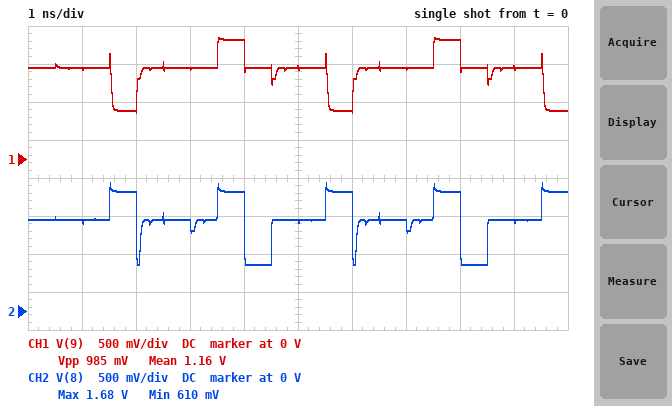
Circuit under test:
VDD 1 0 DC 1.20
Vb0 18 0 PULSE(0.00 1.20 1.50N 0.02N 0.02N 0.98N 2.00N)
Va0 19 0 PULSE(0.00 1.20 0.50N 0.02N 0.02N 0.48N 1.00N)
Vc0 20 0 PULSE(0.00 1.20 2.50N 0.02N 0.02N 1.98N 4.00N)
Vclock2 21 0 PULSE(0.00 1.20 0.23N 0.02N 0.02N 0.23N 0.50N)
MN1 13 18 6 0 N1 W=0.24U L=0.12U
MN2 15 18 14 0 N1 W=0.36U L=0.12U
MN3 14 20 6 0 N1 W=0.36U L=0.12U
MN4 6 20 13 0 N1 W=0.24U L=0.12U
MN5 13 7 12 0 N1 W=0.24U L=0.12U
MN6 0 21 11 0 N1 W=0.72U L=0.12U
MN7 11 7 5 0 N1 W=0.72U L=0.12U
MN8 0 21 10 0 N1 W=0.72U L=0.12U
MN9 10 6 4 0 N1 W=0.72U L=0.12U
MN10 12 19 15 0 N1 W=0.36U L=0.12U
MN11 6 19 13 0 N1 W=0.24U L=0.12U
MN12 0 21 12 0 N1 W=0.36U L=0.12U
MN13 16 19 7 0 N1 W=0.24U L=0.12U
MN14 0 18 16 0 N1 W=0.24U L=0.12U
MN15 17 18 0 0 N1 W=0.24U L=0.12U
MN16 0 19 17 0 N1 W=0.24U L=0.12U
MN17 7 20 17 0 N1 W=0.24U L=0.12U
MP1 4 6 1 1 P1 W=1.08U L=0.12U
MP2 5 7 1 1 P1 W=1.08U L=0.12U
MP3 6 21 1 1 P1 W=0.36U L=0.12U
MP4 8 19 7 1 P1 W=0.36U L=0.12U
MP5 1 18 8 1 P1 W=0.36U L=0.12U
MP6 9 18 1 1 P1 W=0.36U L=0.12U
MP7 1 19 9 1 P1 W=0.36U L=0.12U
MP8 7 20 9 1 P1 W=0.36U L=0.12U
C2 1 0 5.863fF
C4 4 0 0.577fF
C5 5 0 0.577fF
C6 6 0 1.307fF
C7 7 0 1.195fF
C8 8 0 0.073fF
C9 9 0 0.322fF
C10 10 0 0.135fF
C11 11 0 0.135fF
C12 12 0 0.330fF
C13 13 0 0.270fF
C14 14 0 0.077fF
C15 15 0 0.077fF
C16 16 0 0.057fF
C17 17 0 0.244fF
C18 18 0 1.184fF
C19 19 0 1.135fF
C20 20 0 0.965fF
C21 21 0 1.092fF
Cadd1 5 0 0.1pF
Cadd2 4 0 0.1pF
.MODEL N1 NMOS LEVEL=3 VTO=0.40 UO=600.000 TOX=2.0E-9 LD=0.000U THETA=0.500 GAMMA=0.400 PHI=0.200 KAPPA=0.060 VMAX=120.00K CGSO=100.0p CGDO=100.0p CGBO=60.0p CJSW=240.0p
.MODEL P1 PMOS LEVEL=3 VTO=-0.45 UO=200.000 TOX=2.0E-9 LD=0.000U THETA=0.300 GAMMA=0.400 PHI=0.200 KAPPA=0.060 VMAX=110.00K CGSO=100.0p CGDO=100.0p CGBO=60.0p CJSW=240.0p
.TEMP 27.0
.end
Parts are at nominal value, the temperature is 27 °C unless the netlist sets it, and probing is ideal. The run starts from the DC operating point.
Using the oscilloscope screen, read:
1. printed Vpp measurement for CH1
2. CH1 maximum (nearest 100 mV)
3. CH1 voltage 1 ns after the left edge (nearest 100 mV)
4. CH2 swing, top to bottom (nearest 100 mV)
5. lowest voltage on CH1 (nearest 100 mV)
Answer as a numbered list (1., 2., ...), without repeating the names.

1. 985 mV
2. 1.6 V
3. 1.2 V
4. 1.1 V
5. 600 mV
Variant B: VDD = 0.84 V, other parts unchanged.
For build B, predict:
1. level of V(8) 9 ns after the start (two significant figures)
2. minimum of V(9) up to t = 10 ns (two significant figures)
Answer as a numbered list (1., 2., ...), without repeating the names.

1. 840 mV
2. 520 mV
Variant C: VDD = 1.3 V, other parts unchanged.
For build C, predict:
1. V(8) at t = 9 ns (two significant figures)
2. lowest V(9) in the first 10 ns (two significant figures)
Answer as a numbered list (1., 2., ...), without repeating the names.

1. 1.3 V
2. 630 mV
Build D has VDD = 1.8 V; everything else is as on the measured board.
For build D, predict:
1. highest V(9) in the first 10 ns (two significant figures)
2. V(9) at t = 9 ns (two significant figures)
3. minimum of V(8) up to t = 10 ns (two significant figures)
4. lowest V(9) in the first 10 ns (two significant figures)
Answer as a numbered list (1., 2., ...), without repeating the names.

1. 1.9 V
2. 1.8 V
3. 840 mV
4. 900 mV
